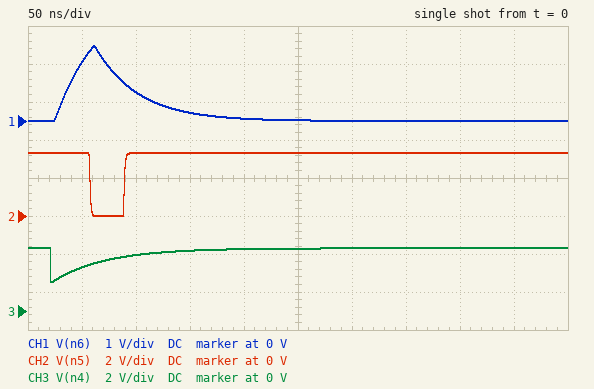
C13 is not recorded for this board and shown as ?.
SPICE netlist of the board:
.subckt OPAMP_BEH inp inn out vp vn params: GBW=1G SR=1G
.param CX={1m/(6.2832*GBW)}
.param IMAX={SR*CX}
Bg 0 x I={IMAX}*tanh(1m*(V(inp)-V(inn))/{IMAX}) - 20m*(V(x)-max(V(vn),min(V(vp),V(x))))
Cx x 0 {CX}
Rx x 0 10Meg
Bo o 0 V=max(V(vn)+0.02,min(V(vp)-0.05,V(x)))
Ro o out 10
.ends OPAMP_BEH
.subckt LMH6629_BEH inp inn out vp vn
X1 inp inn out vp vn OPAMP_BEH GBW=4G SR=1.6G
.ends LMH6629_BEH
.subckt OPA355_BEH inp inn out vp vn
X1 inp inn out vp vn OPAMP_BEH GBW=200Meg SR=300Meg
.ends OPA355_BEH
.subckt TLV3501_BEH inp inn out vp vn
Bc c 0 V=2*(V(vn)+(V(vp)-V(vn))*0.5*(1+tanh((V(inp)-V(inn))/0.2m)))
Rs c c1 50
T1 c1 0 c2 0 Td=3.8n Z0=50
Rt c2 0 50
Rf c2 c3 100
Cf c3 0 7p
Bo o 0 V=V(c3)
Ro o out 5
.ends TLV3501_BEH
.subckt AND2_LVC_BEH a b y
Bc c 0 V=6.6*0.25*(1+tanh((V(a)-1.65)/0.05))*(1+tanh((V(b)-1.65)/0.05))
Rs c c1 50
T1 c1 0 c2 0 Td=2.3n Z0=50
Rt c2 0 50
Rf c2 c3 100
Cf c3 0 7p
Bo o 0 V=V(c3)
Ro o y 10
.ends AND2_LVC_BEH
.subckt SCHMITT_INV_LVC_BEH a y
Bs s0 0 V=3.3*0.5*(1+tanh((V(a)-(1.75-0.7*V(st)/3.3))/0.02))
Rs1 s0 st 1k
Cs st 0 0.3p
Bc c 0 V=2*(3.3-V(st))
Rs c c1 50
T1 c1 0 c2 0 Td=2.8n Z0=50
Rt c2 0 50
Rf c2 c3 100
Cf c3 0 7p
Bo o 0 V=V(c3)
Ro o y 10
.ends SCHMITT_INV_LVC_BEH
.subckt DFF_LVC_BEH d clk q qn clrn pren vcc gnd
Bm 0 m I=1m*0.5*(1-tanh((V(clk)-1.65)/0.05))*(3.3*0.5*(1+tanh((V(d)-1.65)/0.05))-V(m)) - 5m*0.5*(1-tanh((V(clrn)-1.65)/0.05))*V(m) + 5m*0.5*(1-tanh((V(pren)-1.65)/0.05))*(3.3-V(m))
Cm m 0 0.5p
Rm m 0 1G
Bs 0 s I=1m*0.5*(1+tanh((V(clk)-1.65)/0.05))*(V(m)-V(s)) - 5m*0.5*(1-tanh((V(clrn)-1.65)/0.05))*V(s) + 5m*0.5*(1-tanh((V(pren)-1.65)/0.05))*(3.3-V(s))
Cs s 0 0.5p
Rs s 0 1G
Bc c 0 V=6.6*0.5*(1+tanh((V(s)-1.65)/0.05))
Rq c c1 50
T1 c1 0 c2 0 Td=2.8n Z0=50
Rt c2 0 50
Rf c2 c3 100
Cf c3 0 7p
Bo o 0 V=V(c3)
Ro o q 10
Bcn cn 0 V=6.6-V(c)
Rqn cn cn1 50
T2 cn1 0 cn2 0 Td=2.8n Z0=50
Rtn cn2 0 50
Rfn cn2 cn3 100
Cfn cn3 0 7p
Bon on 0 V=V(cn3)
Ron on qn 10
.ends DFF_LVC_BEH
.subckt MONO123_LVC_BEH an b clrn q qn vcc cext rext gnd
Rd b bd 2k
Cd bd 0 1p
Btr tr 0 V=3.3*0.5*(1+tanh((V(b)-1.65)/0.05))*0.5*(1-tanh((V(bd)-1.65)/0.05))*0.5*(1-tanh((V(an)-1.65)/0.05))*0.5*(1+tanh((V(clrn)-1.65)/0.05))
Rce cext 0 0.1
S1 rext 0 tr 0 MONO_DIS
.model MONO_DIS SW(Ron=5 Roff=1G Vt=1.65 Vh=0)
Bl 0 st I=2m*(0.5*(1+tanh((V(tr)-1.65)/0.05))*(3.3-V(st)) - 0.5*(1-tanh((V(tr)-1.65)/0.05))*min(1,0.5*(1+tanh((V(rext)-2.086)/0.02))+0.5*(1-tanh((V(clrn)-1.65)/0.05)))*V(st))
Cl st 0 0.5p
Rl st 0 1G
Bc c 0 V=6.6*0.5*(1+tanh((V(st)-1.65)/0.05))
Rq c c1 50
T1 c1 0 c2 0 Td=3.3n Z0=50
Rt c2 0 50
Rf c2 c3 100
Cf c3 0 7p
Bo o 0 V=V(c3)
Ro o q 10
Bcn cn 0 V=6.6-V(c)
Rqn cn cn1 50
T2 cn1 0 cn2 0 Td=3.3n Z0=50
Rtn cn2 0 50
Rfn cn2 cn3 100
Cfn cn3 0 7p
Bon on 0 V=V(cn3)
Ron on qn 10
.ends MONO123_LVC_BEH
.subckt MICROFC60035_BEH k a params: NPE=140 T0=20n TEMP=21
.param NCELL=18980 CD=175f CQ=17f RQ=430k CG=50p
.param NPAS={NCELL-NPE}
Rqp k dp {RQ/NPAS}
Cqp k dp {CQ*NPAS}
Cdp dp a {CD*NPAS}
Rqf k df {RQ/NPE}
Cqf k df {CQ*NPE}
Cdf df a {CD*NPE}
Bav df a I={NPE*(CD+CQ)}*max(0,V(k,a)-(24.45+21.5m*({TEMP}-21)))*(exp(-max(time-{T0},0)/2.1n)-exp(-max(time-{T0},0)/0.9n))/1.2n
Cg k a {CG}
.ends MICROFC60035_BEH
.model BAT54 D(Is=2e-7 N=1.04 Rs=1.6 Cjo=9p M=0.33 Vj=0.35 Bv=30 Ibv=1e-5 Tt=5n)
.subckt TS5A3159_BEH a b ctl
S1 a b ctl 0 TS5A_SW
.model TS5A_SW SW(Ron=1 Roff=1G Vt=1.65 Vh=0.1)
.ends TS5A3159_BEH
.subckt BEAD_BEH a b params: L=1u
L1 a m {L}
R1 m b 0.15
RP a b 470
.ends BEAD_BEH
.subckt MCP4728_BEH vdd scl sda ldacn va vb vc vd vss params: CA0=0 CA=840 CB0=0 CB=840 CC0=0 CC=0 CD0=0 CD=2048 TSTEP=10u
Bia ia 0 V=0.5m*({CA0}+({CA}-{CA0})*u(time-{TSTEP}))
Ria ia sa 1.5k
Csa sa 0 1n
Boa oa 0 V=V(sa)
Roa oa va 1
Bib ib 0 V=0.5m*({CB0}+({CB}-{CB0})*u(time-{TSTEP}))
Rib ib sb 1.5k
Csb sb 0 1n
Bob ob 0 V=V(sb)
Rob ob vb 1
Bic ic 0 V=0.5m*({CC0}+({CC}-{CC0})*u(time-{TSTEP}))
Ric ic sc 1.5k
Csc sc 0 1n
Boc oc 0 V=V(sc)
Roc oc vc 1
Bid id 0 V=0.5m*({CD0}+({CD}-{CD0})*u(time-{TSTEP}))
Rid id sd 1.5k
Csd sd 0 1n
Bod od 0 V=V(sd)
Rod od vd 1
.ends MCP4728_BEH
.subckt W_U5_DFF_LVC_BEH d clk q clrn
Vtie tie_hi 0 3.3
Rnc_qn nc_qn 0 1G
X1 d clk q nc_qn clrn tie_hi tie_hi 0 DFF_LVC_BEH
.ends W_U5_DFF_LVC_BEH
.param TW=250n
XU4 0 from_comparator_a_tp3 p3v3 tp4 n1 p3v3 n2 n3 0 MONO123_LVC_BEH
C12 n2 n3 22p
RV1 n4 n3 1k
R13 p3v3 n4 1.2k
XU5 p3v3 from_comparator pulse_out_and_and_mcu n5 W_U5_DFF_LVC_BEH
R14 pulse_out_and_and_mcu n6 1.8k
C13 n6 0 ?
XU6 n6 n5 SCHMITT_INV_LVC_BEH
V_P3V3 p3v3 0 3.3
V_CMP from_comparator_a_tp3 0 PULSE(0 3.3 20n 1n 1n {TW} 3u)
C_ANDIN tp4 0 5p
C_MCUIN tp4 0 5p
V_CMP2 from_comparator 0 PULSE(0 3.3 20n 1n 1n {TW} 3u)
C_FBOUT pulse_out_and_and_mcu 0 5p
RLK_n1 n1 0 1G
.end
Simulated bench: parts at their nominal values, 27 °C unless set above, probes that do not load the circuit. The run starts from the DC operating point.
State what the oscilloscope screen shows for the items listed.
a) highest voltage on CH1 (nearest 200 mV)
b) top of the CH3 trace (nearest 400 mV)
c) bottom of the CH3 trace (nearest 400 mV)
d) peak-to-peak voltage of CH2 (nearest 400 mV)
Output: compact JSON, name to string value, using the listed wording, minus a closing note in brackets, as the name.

{"highest voltage on CH1": "2.0 V", "top of the CH3 trace": "3.2 V", "bottom of the CH3 trace": "1.6 V", "peak-to-peak voltage of CH2": "3.2 V"}
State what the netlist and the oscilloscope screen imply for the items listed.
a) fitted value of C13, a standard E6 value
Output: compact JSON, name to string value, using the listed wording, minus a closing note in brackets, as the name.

{"fitted value of C13, a standard E6 value": "22 pF"}
